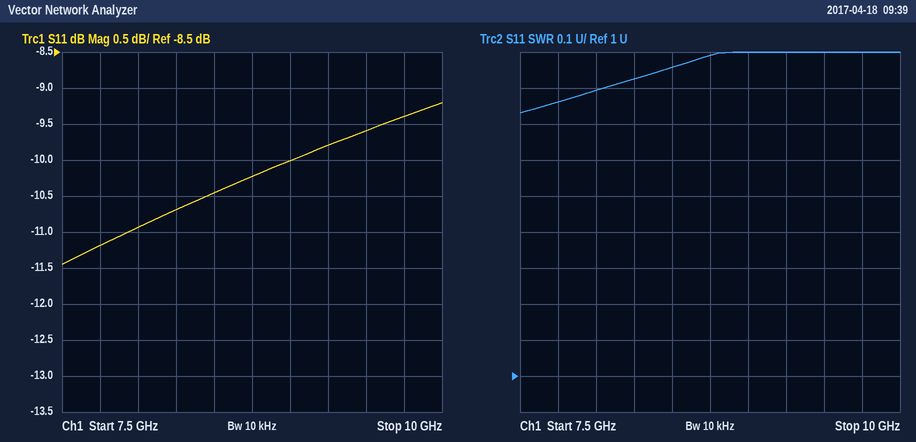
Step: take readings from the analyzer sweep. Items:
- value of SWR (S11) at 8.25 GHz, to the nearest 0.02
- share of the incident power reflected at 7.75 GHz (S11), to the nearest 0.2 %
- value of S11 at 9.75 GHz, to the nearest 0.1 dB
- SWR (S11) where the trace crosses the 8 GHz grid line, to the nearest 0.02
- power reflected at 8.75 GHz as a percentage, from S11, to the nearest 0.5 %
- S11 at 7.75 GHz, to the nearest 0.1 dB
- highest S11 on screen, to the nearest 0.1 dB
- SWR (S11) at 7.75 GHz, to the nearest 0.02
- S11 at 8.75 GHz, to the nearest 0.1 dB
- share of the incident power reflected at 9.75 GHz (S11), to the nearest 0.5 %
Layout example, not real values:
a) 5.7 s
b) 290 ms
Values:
a) 1.82
b) 7.6 %
c) -9.4 dB
d) 1.80
e) 9.5 %
f) -11.2 dB
g) -9.2 dB
h) 1.76
i) -10.2 dB
j) 11.5 %
